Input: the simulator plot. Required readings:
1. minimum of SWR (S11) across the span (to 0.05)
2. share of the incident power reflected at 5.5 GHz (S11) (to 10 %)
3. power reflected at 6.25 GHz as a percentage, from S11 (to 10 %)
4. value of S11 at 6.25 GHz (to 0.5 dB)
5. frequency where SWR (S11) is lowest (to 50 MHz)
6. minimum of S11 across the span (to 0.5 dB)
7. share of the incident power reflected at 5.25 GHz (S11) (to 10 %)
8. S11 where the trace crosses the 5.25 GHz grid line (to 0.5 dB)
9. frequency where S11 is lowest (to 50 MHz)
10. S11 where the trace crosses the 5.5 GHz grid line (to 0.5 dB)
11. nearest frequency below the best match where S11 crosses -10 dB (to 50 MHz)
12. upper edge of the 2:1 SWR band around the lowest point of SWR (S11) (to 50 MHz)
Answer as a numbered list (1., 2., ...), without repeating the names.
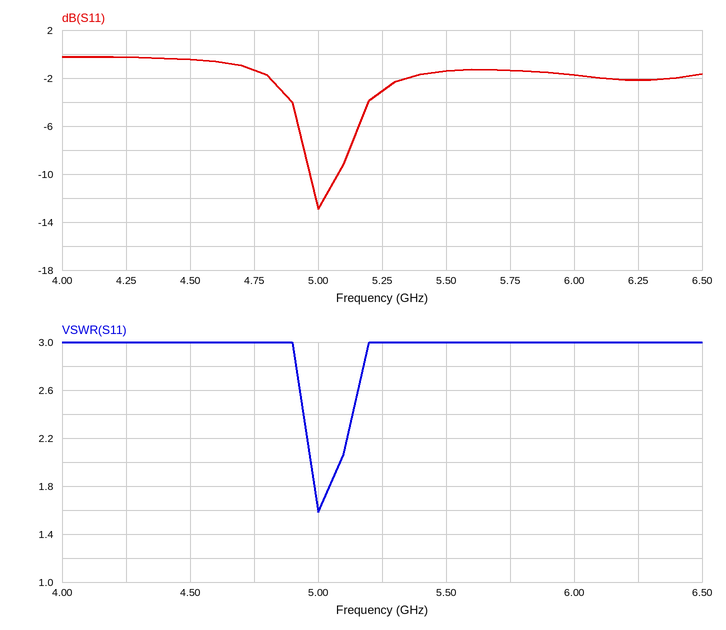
1. 1.60
2. 70 %
3. 60 %
4. -2.0 dB
5. 5.00 GHz
6. -13.0 dB
7. 50 %
8. -3.0 dB
9. 5.00 GHz
10. -1.5 dB
11. 4.95 GHz
12. 5.10 GHz
